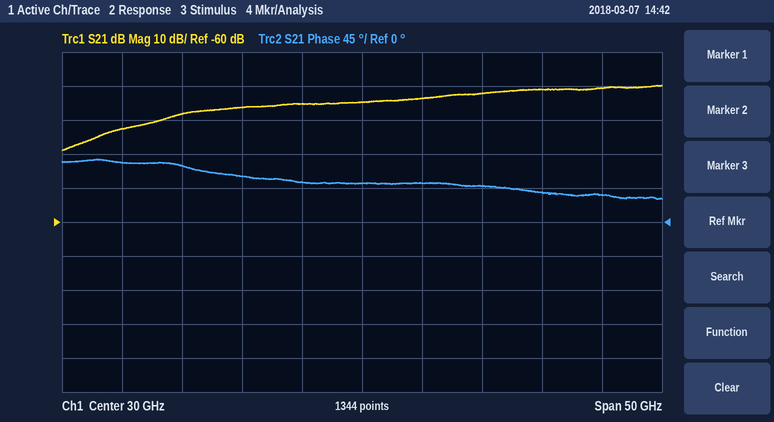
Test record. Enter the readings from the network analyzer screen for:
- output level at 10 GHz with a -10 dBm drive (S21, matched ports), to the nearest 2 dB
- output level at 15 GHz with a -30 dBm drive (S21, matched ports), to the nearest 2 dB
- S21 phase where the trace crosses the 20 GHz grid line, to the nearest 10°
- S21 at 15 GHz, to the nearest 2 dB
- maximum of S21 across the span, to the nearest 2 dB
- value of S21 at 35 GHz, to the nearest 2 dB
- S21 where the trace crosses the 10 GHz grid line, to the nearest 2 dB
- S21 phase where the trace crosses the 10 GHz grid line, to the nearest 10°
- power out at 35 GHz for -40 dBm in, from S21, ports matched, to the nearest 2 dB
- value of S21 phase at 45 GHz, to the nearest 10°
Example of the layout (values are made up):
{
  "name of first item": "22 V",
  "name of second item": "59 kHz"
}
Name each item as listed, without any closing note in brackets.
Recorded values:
{
  "output level at 10 GHz with a -10 dBm drive (S21, matched ports), to the nearest 2 dB": "-42 dBm",
  "output level at 15 GHz with a -30 dBm drive (S21, matched ports), to the nearest 2 dB": "-58 dBm",
  "S21 phase where the trace crosses the 20 GHz grid line, to the nearest 10°": "60°",
  "S21 at 15 GHz, to the nearest 2 dB": "-28 dB",
  "maximum of S21 across the span, to the nearest 2 dB": "-20 dB",
  "value of S21 at 35 GHz, to the nearest 2 dB": "-24 dB",
  "S21 where the trace crosses the 10 GHz grid line, to the nearest 2 dB": "-32 dB",
  "S21 phase where the trace crosses the 10 GHz grid line, to the nearest 10°": "80°",
  "power out at 35 GHz for -40 dBm in, from S21, ports matched, to the nearest 2 dB": "-64 dBm",
  "value of S21 phase at 45 GHz, to the nearest 10°": "40°"
}
